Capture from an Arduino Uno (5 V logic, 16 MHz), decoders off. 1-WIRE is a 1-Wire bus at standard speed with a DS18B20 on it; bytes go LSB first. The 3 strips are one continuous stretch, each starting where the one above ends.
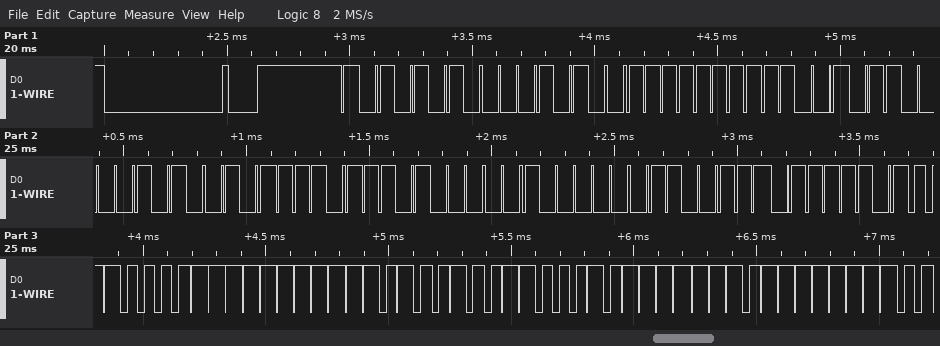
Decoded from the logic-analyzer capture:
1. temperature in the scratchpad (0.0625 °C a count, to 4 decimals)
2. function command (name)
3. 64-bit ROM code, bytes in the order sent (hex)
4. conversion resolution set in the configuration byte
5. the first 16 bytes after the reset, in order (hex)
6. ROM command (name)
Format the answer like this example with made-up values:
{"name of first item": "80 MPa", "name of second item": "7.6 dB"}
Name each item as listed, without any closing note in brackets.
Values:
{"temperature in the scratchpad": "-7.7500 °C", "function command": "Read Scratchpad", "64-bit ROM code, bytes in the order sent": "28 FF D3 50 7A 17 04 E6", "conversion resolution set in the configuration byte": "12 bits", "the first 16 bytes after the reset, in order": "55 28 FF D3 50 7A 17 04 E6 BE 84 FF 4B 46 7F FF", "ROM command": "Match ROM"}
